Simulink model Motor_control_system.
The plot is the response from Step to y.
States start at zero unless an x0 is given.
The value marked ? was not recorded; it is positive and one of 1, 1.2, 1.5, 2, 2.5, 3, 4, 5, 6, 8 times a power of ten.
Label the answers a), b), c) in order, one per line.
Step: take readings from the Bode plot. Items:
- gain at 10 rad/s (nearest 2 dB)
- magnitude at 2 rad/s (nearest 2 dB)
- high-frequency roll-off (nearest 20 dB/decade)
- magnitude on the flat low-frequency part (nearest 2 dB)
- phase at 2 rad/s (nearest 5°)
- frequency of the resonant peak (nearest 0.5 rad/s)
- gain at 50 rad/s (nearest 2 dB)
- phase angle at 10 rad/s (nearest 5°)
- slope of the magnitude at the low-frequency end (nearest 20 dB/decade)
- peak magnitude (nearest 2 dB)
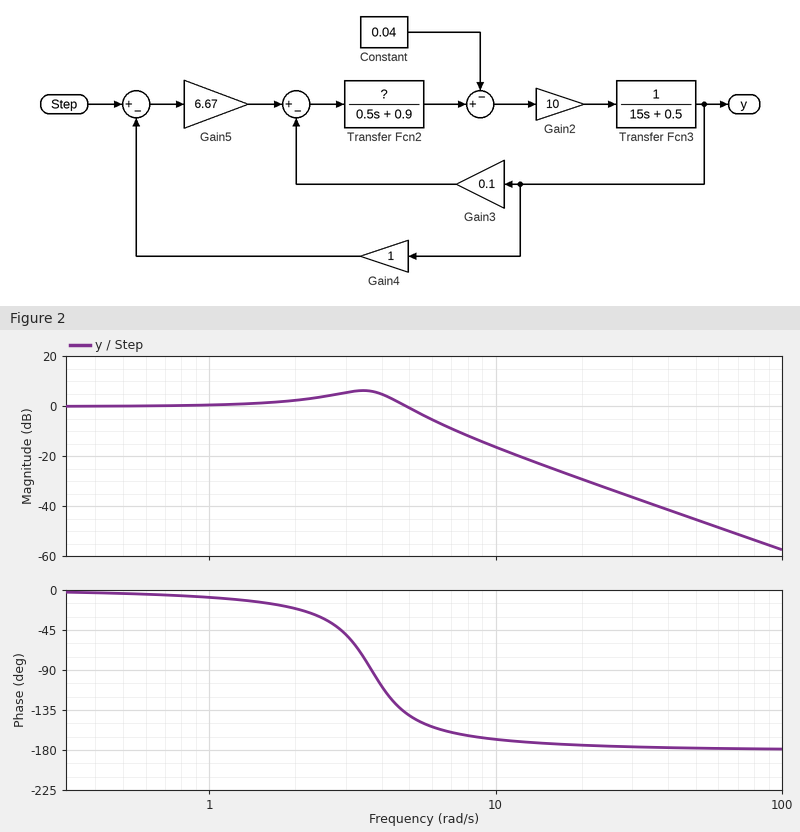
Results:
a) -16 dB
b) 2 dB
c) -40 dB/decade
d) 0 dB
e) -20°
f) 3.5 rad/s
g) -46 dB
h) -170°
i) 0 dB/decade
j) 6 dB
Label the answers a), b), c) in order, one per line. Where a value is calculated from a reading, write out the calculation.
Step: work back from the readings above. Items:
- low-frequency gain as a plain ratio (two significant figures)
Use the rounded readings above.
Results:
a) 10^(0 / 20) = 1.0
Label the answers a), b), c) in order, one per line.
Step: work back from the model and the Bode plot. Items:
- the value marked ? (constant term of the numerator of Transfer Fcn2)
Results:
a) 1.5
